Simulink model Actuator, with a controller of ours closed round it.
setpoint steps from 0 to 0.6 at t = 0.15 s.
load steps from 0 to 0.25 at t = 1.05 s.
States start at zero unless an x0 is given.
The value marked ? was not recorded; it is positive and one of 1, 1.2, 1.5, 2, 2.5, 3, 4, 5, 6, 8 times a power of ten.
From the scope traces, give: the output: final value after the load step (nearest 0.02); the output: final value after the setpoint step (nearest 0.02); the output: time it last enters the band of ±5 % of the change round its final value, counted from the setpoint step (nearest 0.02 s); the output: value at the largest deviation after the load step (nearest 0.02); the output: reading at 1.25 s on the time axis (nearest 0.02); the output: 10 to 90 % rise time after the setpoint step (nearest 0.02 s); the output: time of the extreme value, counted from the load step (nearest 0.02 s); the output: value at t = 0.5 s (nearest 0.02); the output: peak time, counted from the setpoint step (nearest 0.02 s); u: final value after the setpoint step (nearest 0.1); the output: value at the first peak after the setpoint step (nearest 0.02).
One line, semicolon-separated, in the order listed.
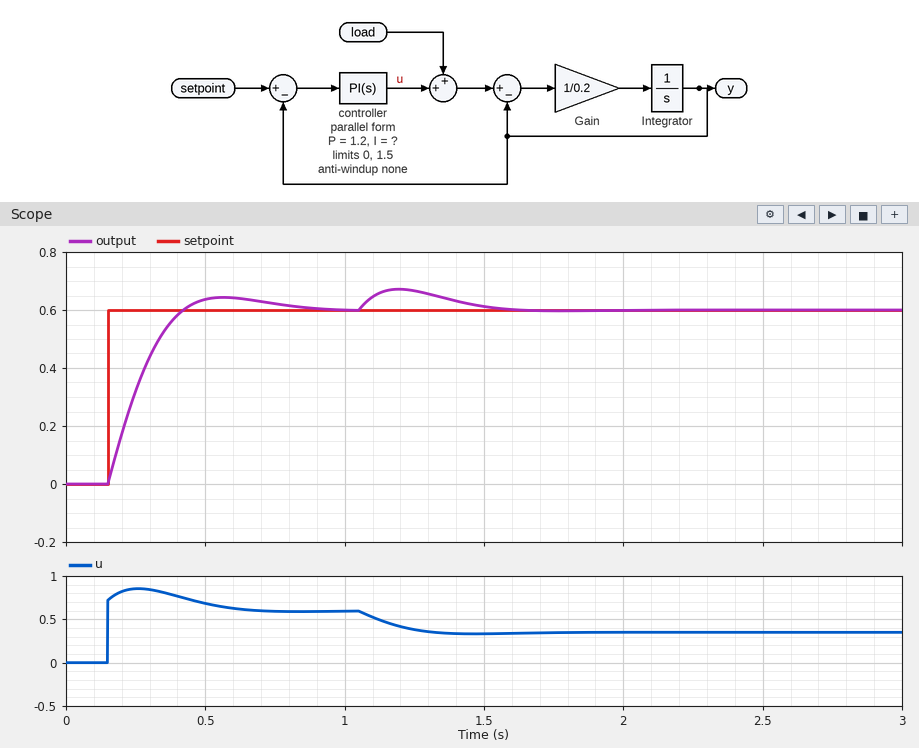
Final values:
0.60; 0.60; 0.54 s; 0.68; 0.66; 0.20 s; 0.14 s; 0.64; 0.42 s; 0.6; 0.64
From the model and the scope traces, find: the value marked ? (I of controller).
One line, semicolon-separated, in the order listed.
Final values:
12
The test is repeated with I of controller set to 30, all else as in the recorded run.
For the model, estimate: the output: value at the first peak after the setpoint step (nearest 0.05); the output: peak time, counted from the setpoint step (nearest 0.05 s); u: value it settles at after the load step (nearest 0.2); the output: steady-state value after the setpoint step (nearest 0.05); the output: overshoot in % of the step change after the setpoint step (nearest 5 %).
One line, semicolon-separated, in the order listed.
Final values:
0.75; 0.25 s; 0.4; 0.60; 25 %
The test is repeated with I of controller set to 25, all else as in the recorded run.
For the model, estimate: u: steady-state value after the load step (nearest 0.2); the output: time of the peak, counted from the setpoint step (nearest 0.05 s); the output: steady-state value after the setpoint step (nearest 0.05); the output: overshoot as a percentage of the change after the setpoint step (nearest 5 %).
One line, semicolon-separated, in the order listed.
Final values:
0.4; 0.25 s; 0.60; 20 %
